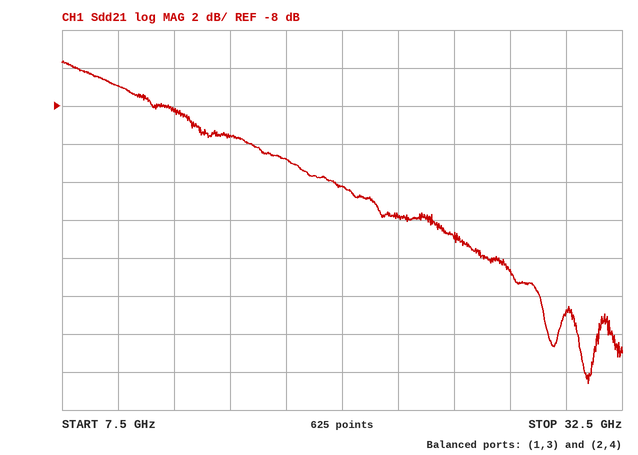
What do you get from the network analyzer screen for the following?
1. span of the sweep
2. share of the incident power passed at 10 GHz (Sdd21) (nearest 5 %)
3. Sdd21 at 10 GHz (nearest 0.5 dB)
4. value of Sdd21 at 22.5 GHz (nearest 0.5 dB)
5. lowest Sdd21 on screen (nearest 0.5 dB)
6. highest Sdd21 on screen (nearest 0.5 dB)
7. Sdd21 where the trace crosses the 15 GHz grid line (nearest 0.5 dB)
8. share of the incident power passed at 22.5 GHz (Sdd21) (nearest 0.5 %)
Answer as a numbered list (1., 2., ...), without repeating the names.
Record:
1. 25 GHz
2. 20 %
3. -7.0 dB
4. -14.0 dB
5. -22.5 dB
6. -5.5 dB
7. -9.5 dB
8. 4.0 %
